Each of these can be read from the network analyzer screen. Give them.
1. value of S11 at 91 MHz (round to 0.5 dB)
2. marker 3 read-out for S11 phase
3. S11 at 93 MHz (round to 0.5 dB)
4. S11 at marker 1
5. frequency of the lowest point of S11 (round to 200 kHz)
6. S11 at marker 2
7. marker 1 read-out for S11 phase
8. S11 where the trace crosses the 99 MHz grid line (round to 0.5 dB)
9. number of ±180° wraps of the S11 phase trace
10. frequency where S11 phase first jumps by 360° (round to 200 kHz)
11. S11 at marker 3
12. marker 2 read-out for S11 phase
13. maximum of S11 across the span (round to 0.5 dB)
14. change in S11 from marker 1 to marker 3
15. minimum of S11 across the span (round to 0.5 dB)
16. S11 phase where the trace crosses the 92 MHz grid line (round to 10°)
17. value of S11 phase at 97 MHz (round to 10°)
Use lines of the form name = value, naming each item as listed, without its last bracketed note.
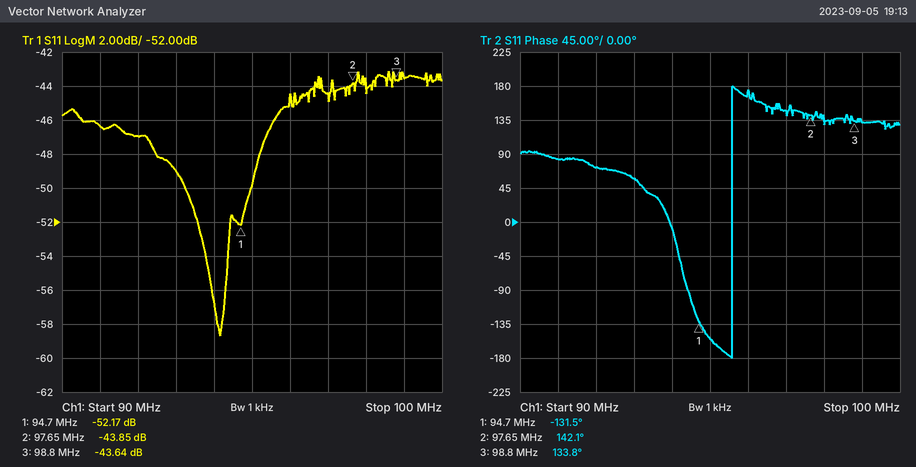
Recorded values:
value of S11 at 91 MHz = -46.5 dB
marker 3 read-out for S11 phase = 133.8°
S11 at 93 MHz = -49.0 dB
S11 at marker 1 = -52.17 dB
frequency of the lowest point of S11 = 94.2 MHz
S11 at marker 2 = -43.85 dB
marker 1 read-out for S11 phase = -131.5°
S11 where the trace crosses the 99 MHz grid line = -43.5 dB
number of ±180° wraps of the S11 phase trace = 1
frequency where S11 phase first jumps by 360° = 95.6 MHz
S11 at marker 3 = -43.64 dB
marker 2 read-out for S11 phase = 142.1°
maximum of S11 across the span = -43.0 dB
change in S11 from marker 1 to marker 3 = 8.53 dB
minimum of S11 across the span = -58.5 dB
S11 phase where the trace crosses the 92 MHz grid line = 70°
value of S11 phase at 97 MHz = 150°
